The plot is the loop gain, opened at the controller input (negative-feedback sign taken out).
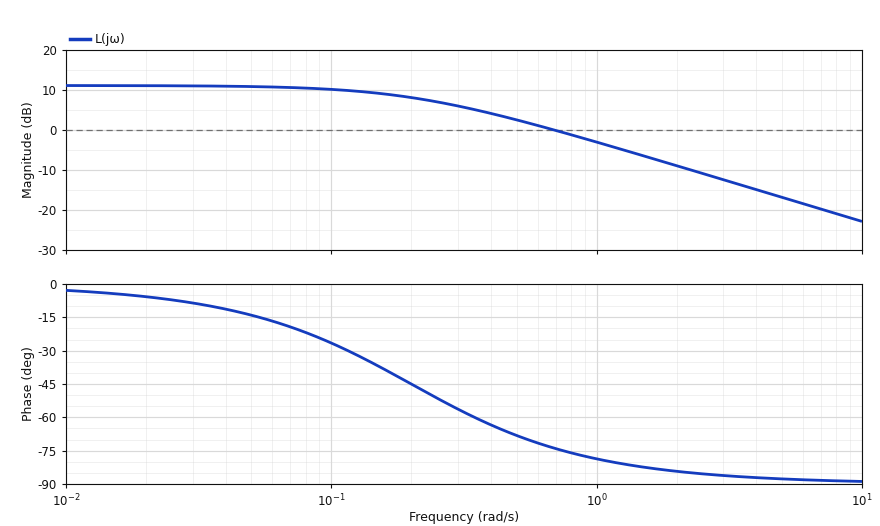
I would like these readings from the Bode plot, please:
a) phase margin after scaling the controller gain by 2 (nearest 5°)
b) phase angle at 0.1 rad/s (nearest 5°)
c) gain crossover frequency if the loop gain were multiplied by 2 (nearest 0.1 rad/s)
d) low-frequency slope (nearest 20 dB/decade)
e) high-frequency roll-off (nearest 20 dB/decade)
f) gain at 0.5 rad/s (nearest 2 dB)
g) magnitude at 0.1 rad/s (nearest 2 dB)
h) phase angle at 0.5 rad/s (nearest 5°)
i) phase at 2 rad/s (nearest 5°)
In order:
100°
-25°
1.4 rad/s
0 dB/decade
-20 dB/decade
2 dB
10 dB
-70°
-85°
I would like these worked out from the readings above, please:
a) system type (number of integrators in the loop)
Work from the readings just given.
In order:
0
